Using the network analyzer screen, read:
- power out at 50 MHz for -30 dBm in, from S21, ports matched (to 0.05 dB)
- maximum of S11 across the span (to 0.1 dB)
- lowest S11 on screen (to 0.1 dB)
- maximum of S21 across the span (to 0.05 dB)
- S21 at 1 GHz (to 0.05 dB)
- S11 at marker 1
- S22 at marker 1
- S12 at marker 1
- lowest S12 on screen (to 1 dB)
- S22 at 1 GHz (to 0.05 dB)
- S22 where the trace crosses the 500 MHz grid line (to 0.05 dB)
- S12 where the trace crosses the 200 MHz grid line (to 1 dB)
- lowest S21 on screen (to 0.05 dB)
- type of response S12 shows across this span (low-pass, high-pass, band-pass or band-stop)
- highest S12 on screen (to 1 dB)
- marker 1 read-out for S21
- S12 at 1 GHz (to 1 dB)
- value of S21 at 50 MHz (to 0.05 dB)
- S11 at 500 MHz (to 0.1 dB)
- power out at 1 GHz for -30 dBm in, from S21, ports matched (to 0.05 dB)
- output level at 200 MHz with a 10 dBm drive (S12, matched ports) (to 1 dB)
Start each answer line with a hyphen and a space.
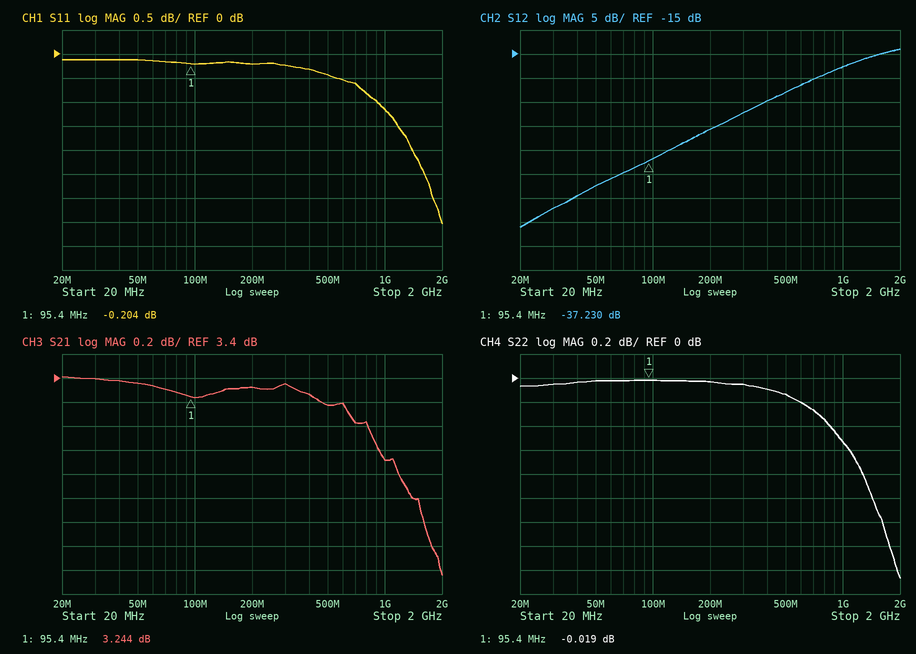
- -26.65 dBm
- -0.1 dB
- -3.5 dB
- 3.40 dB
- 2.70 dB
- -0.204 dB
- -0.019 dB
- -37.230 dB
- -51 dB
- -0.55 dB
- -0.15 dB
- -31 dB
- 1.75 dB
- high-pass
- -14 dB
- 3.244 dB
- -18 dB
- 3.35 dB
- -0.4 dB
- -27.30 dBm
- -21 dBm
